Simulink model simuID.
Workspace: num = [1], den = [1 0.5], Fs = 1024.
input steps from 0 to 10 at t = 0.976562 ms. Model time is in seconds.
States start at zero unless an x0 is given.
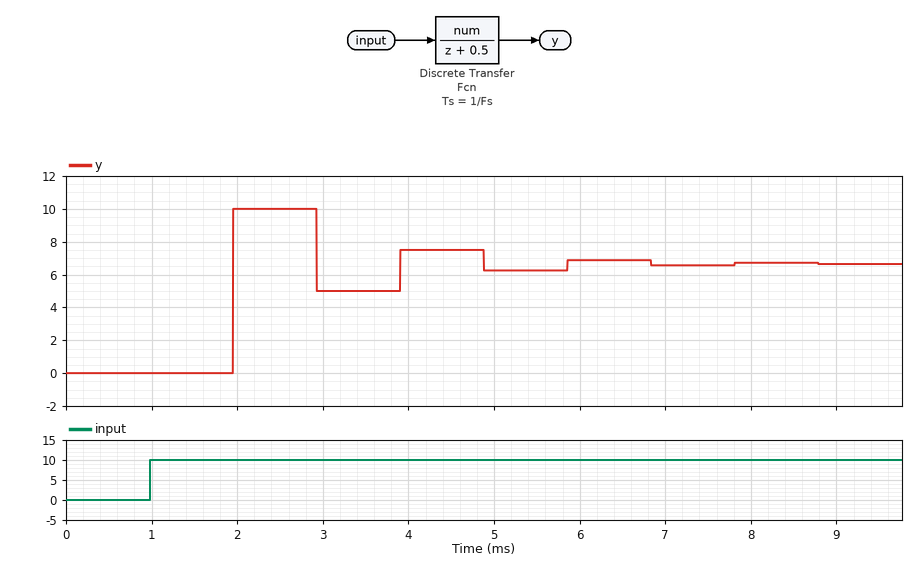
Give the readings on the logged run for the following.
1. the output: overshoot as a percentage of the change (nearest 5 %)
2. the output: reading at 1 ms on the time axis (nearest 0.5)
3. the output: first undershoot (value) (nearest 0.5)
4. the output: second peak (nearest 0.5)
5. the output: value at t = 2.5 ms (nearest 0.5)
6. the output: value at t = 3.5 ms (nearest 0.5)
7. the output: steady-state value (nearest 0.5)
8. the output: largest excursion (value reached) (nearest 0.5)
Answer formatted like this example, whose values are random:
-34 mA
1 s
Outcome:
50 %
0.0
5.0
7.5
10.0
5.0
6.5
10.0
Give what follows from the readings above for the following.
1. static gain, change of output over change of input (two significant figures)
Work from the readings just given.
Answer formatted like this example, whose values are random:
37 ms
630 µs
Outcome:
0.65
